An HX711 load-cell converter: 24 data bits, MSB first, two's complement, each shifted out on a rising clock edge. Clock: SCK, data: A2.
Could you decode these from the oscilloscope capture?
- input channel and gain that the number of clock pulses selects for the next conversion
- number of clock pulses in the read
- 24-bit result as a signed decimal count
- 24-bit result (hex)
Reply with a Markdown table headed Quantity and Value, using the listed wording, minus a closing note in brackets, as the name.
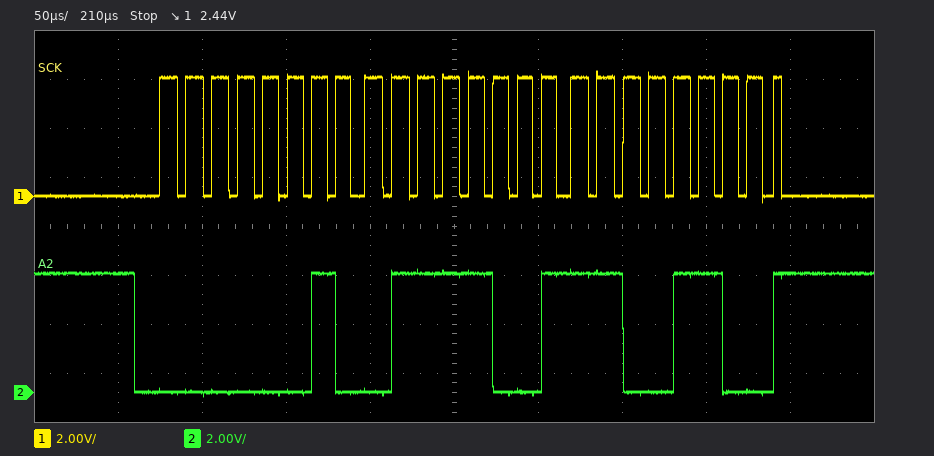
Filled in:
| Quantity | Value |
|---|---|
| input channel and gain that the number of clock pulses selects for the next conversion | channel A, gain 128 |
| number of clock pulses in the read | 25 |
| 24-bit result as a signed decimal count | 162252 |
| 24-bit result | 0x0279CC |
